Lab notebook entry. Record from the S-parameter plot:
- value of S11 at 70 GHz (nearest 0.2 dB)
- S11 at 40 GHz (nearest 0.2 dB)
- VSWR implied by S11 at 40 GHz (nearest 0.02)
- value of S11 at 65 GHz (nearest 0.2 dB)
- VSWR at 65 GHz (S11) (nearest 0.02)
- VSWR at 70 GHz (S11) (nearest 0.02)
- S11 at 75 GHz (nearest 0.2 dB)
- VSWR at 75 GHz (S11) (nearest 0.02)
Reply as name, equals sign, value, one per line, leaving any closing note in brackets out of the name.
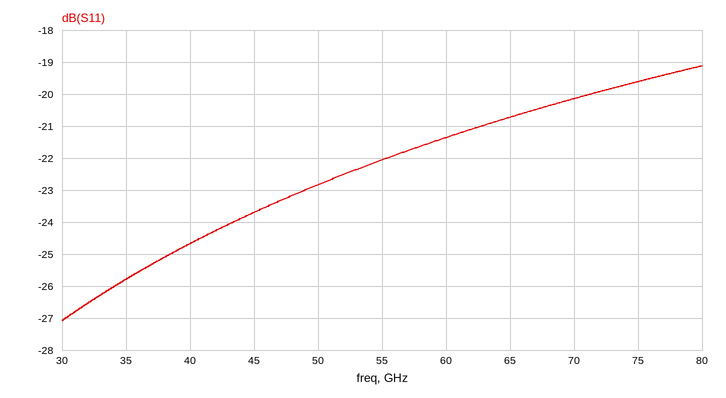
value of S11 at 70 GHz = -20.2 dB
S11 at 40 GHz = -24.6 dB
VSWR implied by S11 at 40 GHz = 1.12
value of S11 at 65 GHz = -20.8 dB
VSWR at 65 GHz (S11) = 1.20
VSWR at 70 GHz (S11) = 1.22
S11 at 75 GHz = -19.6 dB
VSWR at 75 GHz (S11) = 1.24
